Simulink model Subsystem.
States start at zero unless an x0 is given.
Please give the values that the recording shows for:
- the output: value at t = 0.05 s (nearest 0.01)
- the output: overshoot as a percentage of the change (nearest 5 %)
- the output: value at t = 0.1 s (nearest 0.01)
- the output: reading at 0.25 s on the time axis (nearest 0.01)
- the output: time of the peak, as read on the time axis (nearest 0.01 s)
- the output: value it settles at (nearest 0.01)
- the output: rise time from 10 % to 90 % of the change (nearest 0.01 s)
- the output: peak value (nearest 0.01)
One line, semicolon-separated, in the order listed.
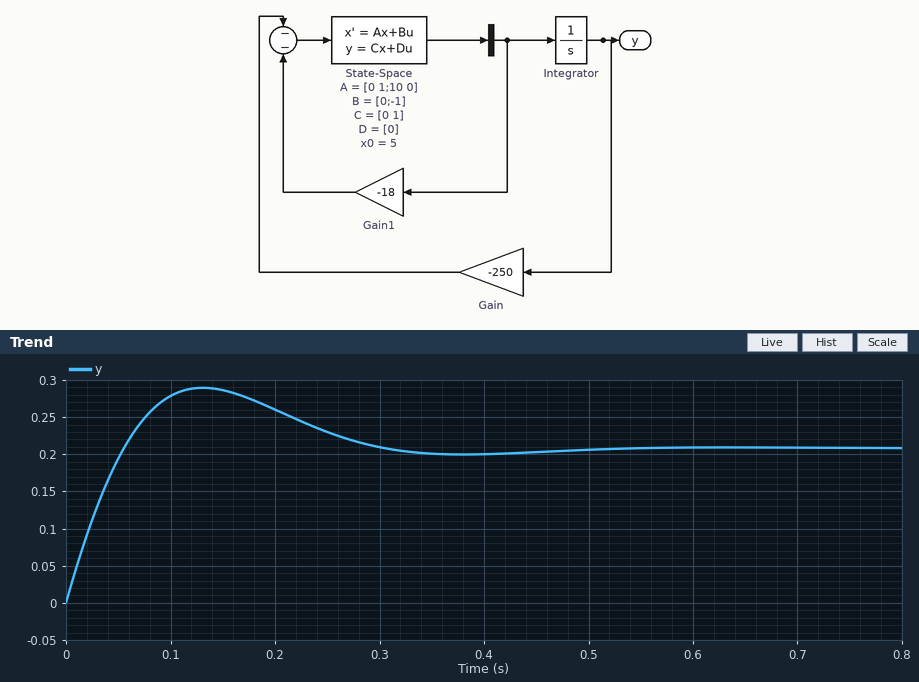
0.19; 40 %; 0.28; 0.23; 0.13 s; 0.21; 0.04 s; 0.29
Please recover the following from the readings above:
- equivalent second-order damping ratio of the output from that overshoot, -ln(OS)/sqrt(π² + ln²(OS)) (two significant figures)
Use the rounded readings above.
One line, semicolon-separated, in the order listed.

0.28
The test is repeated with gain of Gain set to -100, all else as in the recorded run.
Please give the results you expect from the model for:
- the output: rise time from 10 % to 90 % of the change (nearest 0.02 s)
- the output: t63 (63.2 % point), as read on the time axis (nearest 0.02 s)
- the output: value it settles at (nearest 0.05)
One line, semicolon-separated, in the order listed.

0.22 s; 0.10 s; 0.55
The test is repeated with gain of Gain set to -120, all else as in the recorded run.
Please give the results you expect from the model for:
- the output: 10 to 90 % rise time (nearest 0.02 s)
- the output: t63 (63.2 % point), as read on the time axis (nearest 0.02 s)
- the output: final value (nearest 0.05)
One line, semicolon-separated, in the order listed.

0.14 s; 0.08 s; 0.45
